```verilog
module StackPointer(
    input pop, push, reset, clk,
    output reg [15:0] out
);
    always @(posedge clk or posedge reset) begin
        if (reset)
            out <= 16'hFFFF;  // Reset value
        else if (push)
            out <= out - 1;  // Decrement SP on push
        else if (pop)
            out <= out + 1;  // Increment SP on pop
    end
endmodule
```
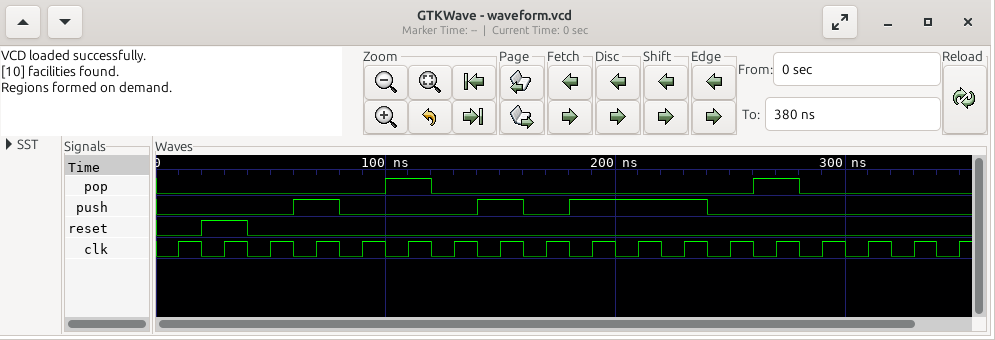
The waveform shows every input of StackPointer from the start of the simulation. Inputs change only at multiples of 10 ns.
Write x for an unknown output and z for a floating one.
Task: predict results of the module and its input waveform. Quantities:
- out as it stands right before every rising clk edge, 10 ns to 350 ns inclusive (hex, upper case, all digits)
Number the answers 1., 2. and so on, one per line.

1. x, FFFF, FFFF, FFFF, FFFE, FFFE, FFFF, FFFF, FFFE, FFFE, FFFD, FFFC, FFFB, FFFB, FFFC, FFFC, FFFC, FFFC
